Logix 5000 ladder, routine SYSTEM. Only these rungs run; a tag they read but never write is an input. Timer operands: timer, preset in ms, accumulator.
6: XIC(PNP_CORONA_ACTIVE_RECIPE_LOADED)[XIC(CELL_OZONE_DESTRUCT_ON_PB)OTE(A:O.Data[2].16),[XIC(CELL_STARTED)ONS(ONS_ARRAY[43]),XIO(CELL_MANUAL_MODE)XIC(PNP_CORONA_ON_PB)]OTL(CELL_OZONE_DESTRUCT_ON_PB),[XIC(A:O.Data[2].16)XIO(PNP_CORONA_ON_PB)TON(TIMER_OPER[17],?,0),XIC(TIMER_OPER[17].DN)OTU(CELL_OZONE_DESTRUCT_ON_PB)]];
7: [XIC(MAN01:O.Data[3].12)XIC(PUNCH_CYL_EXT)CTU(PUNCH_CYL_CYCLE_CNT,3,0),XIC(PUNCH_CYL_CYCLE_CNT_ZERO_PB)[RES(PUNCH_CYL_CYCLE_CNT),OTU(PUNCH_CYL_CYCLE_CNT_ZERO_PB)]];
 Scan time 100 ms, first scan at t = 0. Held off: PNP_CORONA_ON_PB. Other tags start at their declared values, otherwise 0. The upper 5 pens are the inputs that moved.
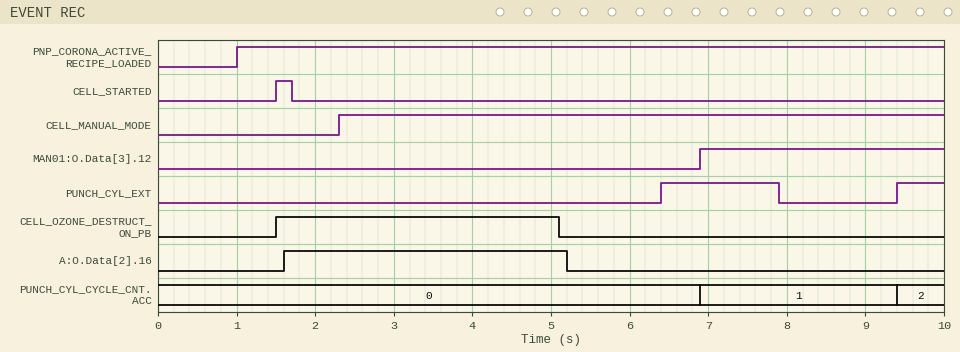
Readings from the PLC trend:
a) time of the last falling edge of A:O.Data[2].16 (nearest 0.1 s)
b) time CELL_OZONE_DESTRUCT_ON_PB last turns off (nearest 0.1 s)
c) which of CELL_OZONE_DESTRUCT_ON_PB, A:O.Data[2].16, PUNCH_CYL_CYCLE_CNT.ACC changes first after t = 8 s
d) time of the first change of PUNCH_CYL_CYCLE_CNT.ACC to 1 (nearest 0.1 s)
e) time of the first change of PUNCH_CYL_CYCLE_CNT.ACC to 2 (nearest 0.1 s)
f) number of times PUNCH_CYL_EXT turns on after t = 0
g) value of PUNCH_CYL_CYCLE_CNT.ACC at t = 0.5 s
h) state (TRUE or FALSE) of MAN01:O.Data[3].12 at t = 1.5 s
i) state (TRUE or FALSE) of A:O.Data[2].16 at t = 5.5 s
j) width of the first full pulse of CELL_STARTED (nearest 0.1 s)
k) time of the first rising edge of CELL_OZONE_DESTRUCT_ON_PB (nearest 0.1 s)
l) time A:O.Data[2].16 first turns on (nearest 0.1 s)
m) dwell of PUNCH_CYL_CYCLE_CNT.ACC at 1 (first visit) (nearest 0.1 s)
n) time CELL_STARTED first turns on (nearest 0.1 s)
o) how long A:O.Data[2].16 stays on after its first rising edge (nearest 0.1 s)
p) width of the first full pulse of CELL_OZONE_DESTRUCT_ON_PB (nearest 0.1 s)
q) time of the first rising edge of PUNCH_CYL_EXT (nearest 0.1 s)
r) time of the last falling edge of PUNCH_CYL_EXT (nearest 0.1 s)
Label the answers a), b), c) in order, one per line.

a) 5.2 s
b) 5.1 s
c) PUNCH_CYL_CYCLE_CNT.ACC
d) 6.9 s
e) 9.4 s
f) 2
g) 0
h) FALSE
i) FALSE
j) 0.2 s
k) 1.5 s
l) 1.6 s
m) 2.5 s
n) 1.5 s
o) 3.6 s
p) 3.6 s
q) 6.4 s
r) 7.9 s
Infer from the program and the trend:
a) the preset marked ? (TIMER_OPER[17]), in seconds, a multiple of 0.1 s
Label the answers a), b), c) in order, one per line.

a) 3.5 s
